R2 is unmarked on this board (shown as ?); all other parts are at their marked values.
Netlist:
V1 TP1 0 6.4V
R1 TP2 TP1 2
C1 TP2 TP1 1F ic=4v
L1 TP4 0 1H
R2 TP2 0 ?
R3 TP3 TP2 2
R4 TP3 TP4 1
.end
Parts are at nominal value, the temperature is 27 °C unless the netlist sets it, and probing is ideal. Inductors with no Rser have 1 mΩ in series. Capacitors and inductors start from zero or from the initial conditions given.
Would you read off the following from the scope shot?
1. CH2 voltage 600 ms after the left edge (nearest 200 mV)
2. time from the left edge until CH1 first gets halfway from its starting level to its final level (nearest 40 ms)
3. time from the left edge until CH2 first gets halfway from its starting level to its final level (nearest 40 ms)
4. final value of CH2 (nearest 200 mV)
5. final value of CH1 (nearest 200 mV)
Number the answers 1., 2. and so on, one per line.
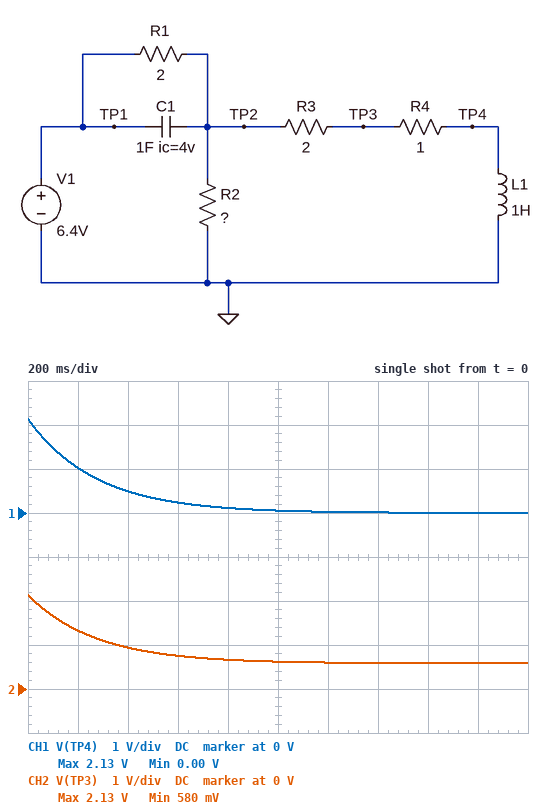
1. 800 mV
2. 200 ms
3. 200 ms
4. 600 mV
5. 0 V
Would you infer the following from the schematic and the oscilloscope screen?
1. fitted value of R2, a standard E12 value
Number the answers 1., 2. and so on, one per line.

1. 1 Ω
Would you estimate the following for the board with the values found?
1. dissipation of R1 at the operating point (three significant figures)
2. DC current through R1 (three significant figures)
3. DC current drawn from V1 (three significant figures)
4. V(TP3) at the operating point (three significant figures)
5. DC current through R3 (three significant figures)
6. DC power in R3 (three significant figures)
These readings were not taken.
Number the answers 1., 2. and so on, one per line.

1. 10.8 W
2. 2.33 A
3. 2.33 A
4. 582 mV
5. 582 mA
6. 677 mW
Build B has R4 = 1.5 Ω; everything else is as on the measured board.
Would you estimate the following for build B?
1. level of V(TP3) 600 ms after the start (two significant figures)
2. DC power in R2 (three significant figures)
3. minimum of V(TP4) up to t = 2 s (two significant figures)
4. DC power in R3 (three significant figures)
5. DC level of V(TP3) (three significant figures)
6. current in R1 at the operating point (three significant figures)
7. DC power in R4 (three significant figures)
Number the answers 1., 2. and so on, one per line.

1. 880 mV
2. 3.21 W
3. 1.0 mV
4. 524 mW
5. 768 mV
6. 2.30 A
7. 393 mW
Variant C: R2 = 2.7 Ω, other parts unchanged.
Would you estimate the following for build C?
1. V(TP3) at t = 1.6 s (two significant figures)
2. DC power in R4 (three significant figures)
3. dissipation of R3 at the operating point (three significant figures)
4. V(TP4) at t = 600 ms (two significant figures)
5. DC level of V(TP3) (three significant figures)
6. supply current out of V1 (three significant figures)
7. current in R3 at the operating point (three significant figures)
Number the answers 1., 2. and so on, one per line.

1. 890 mV
2. 785 mW
3. 1.57 W
4. 310 mV
5. 887 mV
6. 1.87 A
7. 886 mA
